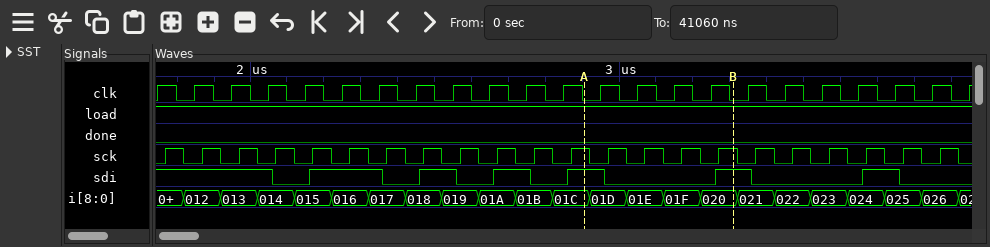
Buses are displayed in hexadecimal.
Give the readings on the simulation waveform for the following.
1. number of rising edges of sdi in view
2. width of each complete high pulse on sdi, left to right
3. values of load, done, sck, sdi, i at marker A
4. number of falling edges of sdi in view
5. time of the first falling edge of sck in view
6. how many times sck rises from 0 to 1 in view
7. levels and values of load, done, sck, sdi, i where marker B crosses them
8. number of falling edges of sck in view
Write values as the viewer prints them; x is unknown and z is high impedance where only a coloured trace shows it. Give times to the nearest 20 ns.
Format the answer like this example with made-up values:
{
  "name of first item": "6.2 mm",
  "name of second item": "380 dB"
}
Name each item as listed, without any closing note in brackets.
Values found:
{
  "number of rising edges of sdi in view": "6",
  "width of each complete high pulse on sdi, left to right": "200 ns, 100 ns, 100 ns, 100 ns, 100 ns, 100 ns",
  "values of load, done, sck, sdi, i at marker A": "load=1, done=0, sck=1, sdi=1, i=01C",
  "number of falling edges of sdi in view": "7",
  "time of the first falling edge of sck in view": "1820 ns",
  "how many times sck rises from 0 to 1 in view": "22",
  "levels and values of load, done, sck, sdi, i where marker B crosses them": "load=1, done=0, sck=1, sdi=1, i=020",
  "number of falling edges of sck in view": "22"
}
